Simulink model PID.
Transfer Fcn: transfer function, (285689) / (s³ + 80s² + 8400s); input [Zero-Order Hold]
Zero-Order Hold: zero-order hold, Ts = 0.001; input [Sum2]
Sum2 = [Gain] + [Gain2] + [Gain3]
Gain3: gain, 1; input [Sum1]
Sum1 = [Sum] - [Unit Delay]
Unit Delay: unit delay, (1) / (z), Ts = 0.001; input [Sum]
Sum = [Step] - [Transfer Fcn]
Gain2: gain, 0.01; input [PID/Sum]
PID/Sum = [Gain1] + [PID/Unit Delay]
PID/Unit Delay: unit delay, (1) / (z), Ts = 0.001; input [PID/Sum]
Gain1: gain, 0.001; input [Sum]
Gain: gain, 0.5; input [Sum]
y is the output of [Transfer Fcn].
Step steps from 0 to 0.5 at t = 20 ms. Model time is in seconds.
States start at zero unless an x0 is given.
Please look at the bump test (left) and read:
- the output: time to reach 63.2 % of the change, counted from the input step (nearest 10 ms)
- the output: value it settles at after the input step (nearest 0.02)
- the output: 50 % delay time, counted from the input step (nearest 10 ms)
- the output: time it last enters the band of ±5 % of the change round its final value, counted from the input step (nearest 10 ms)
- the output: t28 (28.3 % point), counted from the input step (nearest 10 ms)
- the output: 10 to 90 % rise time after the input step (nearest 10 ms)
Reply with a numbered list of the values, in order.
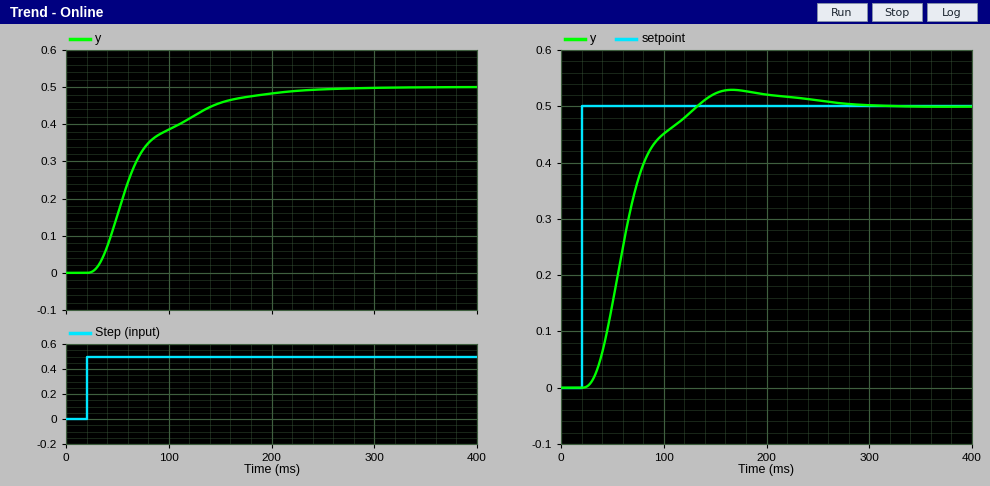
1. 50 ms
2. 0.50
3. 40 ms
4. 160 ms
5. 30 ms
6. 110 ms
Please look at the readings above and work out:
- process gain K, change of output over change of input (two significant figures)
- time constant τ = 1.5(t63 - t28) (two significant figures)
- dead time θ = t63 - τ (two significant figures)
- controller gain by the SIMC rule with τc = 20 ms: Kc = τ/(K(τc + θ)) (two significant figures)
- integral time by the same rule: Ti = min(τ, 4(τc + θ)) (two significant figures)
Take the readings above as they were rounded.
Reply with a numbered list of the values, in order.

1. 1.0
2. 30 ms
3. 20 ms
4. 0.75
5. 30 ms
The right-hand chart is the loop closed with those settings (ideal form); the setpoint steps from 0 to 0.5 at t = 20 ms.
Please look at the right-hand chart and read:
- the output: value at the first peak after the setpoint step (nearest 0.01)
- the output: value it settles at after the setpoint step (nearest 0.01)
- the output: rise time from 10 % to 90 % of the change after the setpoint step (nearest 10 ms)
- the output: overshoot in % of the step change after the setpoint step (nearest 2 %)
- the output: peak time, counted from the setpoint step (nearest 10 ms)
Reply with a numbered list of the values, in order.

1. 0.53
2. 0.50
3. 60 ms
4. 6 %
5. 150 ms
